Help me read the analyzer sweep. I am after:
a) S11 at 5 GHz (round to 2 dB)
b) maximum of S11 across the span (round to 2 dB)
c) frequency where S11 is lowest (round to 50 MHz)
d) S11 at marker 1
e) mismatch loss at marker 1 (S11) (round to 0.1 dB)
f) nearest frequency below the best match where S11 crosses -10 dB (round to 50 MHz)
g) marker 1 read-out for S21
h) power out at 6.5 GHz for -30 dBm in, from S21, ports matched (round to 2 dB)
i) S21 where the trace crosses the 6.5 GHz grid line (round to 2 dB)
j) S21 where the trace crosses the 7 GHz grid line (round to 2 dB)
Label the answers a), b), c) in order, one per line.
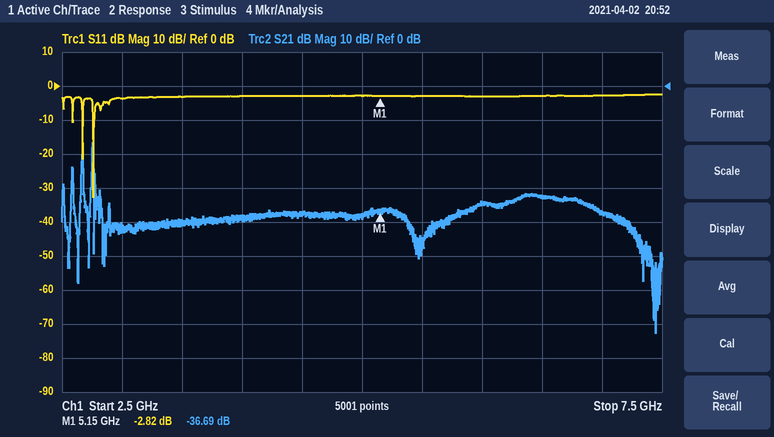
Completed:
a) -2 dB
b) -2 dB
c) 2.75 GHz
d) -2.82 dB
e) 3.2 dB
f) 2.75 GHz
g) -36.69 dB
h) -62 dBm
i) -32 dB
j) -38 dB
